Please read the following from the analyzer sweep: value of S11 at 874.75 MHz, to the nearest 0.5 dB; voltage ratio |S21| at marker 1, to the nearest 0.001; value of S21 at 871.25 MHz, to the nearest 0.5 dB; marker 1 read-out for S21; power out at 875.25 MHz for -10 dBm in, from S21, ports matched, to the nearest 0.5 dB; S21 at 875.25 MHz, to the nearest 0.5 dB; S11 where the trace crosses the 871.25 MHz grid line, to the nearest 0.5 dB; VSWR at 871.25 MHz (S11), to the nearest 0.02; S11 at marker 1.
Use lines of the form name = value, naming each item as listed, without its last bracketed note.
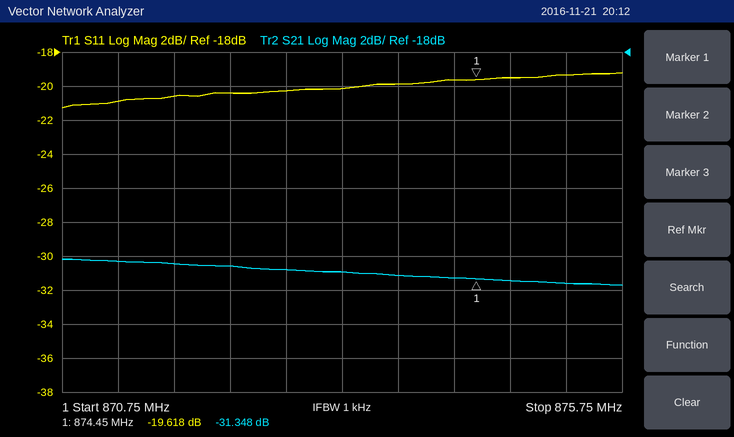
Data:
value of S11 at 874.75 MHz, to the nearest 0.5 dB = -19.5 dB
voltage ratio |S21| at marker 1, to the nearest 0.001 = 0.027
value of S21 at 871.25 MHz, to the nearest 0.5 dB = -30.5 dB
marker 1 read-out for S21 = -31.348 dB
power out at 875.25 MHz for -10 dBm in, from S21, ports matched, to the nearest 0.5 dB = -41.5 dBm
S21 at 875.25 MHz, to the nearest 0.5 dB = -31.5 dB
S11 where the trace crosses the 871.25 MHz grid line, to the nearest 0.5 dB = -21.0 dB
VSWR at 871.25 MHz (S11), to the nearest 0.02 = 1.20
S11 at marker 1 = -19.618 dB
